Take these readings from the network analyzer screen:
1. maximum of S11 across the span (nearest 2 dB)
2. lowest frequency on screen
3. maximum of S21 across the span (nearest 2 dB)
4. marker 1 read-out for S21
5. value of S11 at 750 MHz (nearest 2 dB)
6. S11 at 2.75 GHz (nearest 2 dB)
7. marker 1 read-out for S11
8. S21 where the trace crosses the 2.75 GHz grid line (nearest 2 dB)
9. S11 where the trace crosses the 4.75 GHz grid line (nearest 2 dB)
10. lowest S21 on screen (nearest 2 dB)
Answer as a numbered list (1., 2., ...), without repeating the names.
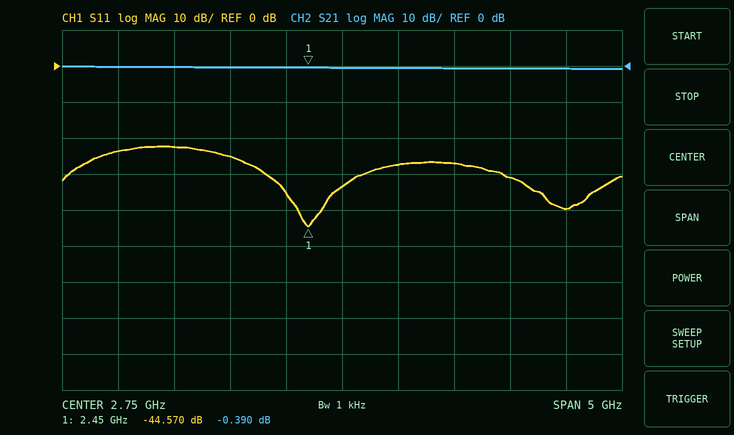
1. -22 dB
2. 250 MHz
3. 0 dB
4. -0.390 dB
5. -24 dB
6. -34 dB
7. -44.570 dB
8. 0 dB
9. -40 dB
10. 0 dB
